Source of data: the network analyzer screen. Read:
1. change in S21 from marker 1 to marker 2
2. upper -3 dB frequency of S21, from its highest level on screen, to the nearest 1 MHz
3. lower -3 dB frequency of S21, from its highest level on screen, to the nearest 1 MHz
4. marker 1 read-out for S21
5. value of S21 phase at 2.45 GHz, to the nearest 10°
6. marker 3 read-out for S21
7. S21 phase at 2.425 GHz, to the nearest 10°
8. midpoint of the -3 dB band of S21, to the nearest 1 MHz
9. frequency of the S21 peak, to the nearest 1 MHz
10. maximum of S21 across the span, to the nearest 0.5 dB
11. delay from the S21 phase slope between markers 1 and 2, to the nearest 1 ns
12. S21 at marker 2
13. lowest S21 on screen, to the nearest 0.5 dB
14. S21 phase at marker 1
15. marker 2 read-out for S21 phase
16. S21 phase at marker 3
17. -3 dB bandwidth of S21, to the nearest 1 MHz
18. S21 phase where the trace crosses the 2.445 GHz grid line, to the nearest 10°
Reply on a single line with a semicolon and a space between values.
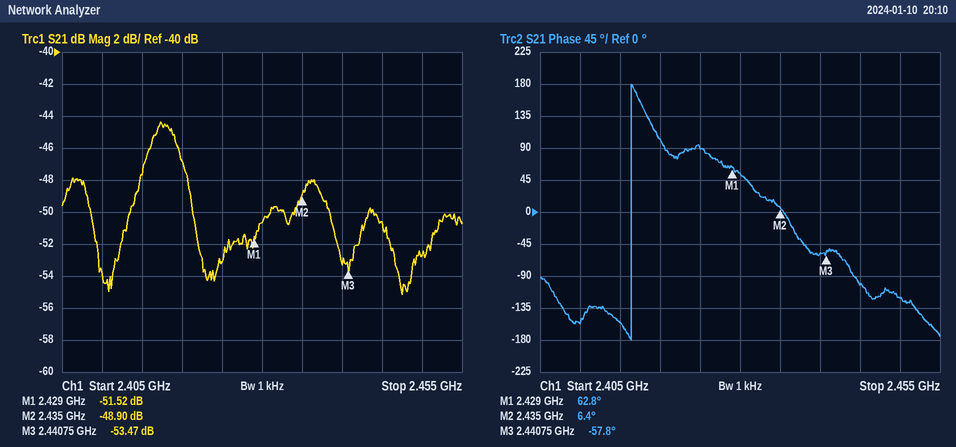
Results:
2.62 dB; 2.420 GHz; 2.415 GHz; -51.52 dB; -120°; -53.47 dB; 90°; 2.418 GHz; 2.417 GHz; -44.5 dB; 26 ns; -48.90 dB; -55.0 dB; 62.8°; 6.4°; -57.8°; 5 MHz; -100°
